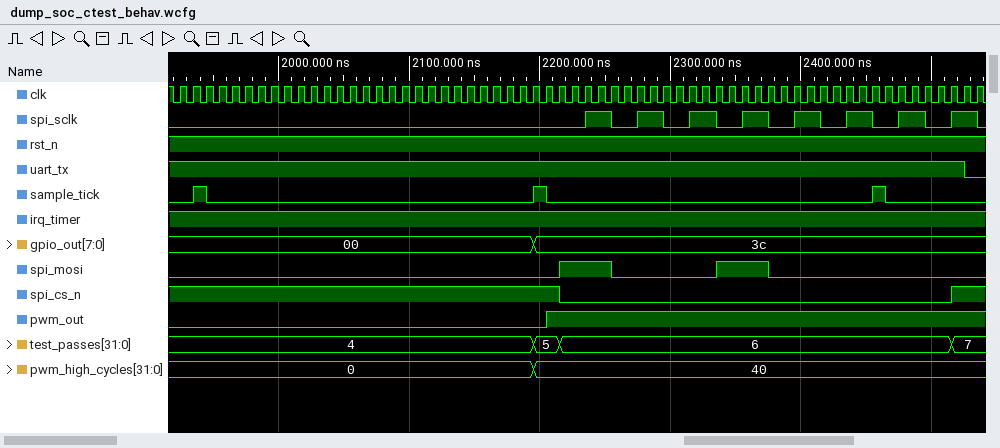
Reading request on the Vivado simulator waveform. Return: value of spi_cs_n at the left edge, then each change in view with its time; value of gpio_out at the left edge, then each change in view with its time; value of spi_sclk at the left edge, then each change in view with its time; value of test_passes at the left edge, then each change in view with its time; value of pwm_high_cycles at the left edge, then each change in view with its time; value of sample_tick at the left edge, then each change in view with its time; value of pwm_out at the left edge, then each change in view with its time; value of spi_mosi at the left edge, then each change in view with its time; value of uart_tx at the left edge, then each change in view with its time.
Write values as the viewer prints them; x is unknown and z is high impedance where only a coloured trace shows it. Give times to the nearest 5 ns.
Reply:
1, 0 at 2215 ns, 1 at 2515 ns
00, 3c at 2195 ns
0, 1 at 2235 ns, 0 at 2255 ns, 1 at 2275 ns, 0 at 2295 ns, 1 at 2315 ns, 0 at 2335 ns, 1 at 2355 ns, 0 at 2375 ns, 1 at 2395 ns, 0 at 2415 ns, 1 at 2435 ns, 0 at 2455 ns, 1 at 2475 ns, 0 at 2495 ns, 1 at 2515 ns, 0 at 2535 ns
4, 5 at 2195 ns, 6 at 2215 ns, 7 at 2515 ns
0, 40 at 2195 ns
0, 1 at 1935 ns, 0 at 1945 ns, 1 at 2195 ns, 0 at 2205 ns, 1 at 2455 ns, 0 at 2465 ns
0, 1 at 2205 ns
0, 1 at 2215 ns, 0 at 2255 ns, 1 at 2335 ns, 0 at 2375 ns
1, 0 at 2525 ns
